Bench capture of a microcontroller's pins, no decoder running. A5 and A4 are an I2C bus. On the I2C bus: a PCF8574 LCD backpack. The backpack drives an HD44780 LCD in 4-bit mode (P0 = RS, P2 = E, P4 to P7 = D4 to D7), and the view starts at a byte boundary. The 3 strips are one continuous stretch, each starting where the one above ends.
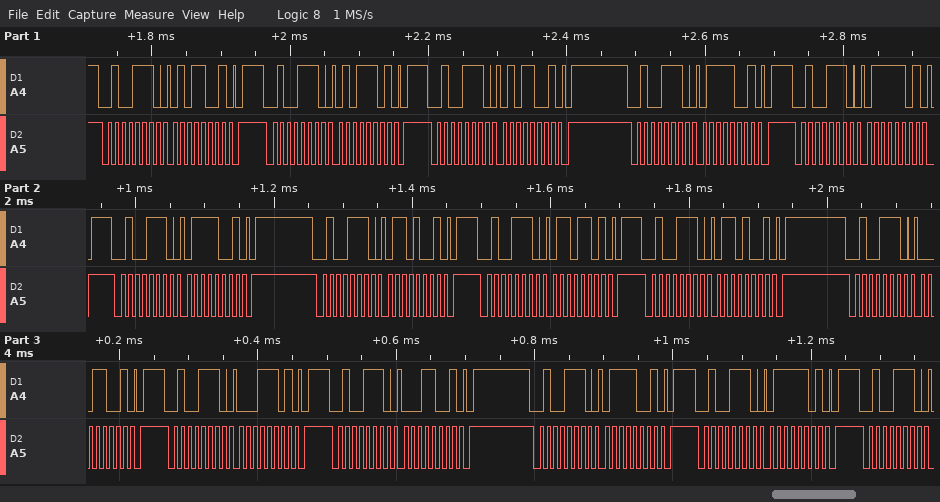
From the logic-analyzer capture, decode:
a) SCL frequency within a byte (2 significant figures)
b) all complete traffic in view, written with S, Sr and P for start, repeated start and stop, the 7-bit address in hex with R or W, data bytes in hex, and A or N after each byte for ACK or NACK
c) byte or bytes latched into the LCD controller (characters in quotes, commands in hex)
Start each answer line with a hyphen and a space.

- 100 kHz
- S 27W A 59 A P S 27W A 5D A P S 27W A 59 A P S 27W A 79 A P S 27W A 7D A P S 27W A 79 A P S 27W A 69 A P S 27W A 6D A P S 27W A 69 A P S 27W A 19 A P S 27W A 1D A P S 27W A 19 A P S 27W A 79 A P S 27W A 7D A P S 27W A
- 'W' 'a'
